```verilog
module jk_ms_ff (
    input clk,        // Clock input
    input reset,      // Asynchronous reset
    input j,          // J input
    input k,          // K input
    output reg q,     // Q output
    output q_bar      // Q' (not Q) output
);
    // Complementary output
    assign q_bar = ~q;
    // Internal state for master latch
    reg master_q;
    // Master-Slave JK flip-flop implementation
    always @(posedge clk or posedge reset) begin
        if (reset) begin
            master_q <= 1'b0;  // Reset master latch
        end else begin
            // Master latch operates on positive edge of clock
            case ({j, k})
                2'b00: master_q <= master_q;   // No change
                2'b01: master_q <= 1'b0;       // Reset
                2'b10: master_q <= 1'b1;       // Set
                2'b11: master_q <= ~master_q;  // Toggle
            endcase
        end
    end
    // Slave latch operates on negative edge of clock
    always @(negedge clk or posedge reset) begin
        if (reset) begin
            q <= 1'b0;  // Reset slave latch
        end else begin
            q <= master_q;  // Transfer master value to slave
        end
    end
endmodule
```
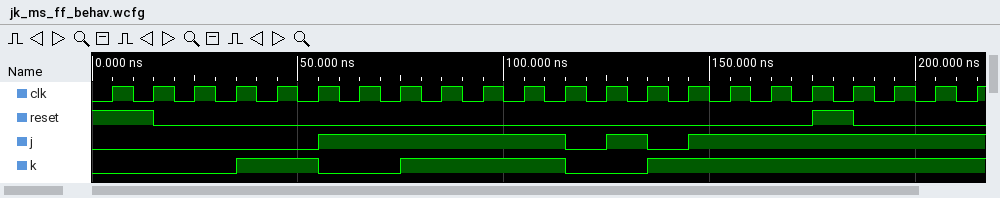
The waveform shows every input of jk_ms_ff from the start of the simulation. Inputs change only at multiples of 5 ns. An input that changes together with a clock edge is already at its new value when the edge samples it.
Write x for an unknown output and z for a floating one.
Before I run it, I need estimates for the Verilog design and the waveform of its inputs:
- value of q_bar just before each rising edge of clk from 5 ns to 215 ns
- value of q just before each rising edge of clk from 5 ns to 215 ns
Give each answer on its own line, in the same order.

1 1 1 1 1 1 0 0 1 0 1 0 0 0 1 0 1 0 1 0 1 0
0 0 0 0 0 0 1 1 0 1 0 1 1 1 0 1 0 1 0 1 0 1
